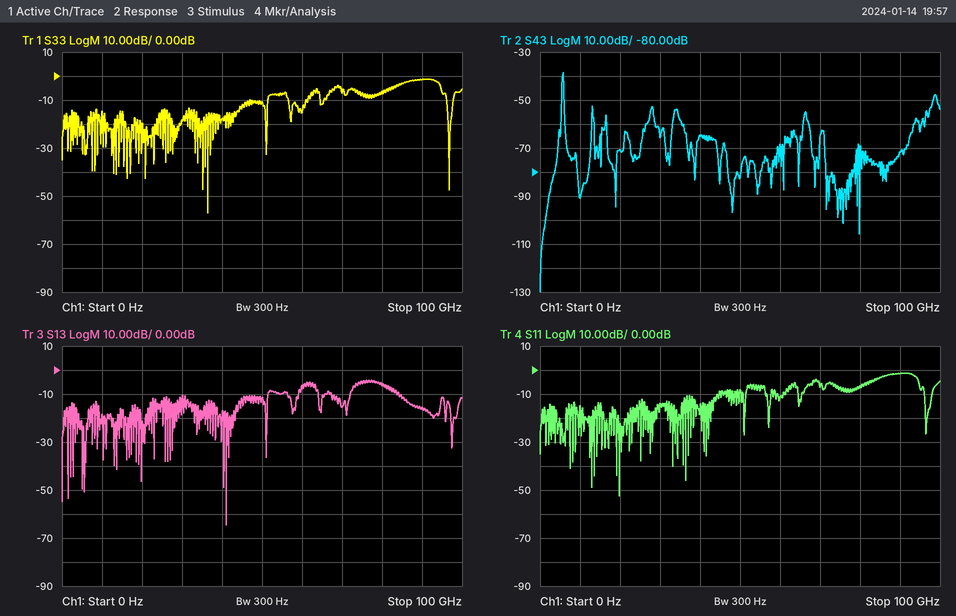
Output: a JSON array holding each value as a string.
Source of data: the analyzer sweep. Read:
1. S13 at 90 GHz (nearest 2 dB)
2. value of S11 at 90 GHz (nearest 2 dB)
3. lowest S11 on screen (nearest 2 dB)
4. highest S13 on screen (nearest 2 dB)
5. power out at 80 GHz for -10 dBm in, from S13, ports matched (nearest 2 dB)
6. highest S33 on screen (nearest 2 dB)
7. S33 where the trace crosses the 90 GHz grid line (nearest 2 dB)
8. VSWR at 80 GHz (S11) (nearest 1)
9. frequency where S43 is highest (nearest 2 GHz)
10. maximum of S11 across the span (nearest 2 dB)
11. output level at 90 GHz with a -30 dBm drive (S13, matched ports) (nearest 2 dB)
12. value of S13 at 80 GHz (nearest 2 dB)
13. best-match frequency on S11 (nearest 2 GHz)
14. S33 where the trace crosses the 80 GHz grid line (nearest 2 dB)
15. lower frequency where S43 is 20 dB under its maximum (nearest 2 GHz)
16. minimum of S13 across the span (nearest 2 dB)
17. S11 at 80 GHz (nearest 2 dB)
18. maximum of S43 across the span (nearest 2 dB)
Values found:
["-16 dB", "-2 dB", "-52 dB", "-4 dB", "-16 dBm", "-2 dB", "-2 dB", "3", "6 GHz", "-2 dB", "-46 dBm", "-6 dB", "20 GHz", "-6 dB", "6 GHz", "-64 dB", "-6 dB", "-38 dB"]
